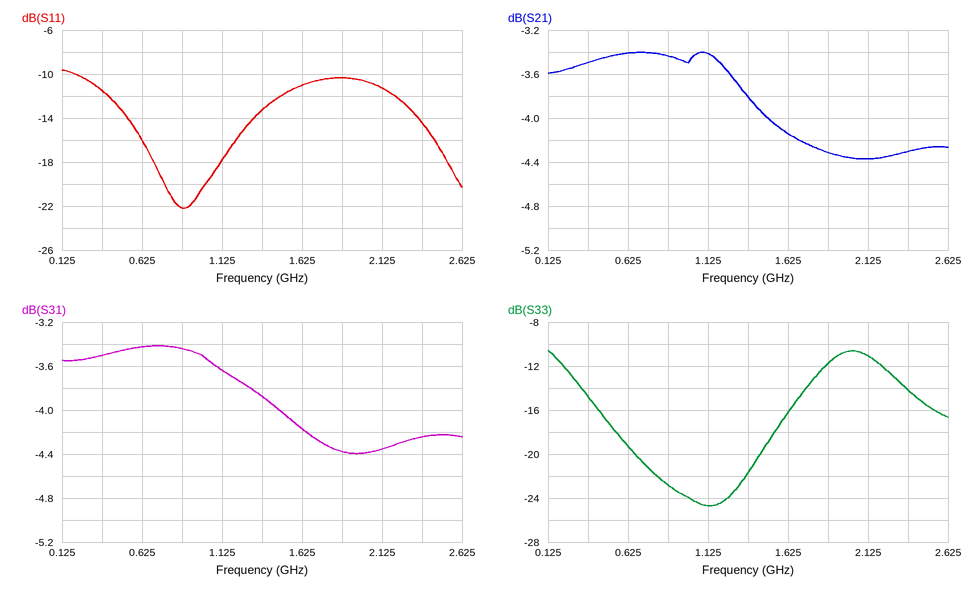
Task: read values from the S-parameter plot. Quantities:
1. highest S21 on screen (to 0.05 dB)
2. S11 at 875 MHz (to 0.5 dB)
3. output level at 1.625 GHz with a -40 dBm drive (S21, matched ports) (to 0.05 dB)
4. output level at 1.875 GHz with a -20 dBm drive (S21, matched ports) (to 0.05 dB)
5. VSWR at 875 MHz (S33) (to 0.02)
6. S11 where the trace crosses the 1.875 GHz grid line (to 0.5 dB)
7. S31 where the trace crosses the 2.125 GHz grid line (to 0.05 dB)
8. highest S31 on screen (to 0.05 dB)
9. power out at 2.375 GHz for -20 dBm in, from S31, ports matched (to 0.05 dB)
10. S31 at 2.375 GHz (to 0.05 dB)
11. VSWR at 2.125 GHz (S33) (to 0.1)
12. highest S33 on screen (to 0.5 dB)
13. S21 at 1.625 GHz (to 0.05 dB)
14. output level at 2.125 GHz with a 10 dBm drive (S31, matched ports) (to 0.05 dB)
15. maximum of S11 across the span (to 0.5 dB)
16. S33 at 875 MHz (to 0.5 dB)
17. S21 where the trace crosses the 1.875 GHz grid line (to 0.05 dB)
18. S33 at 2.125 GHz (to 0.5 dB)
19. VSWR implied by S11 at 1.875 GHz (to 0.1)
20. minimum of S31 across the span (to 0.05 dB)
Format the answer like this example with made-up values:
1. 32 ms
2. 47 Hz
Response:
1. -3.40 dB
2. -22.0 dB
3. -44.15 dBm
4. -24.30 dBm
5. 1.16
6. -10.5 dB
7. -4.35 dB
8. -3.40 dB
9. -24.25 dBm
10. -4.25 dB
11. 1.8
12. -10.5 dB
13. -4.15 dB
14. 5.65 dBm
15. -9.5 dB
16. -23.0 dB
17. -4.30 dB
18. -11.0 dB
19. 1.9
20. -4.40 dB
